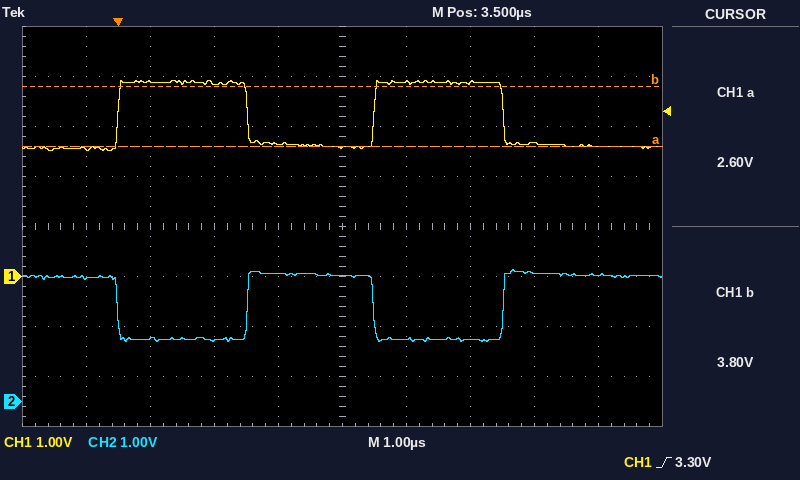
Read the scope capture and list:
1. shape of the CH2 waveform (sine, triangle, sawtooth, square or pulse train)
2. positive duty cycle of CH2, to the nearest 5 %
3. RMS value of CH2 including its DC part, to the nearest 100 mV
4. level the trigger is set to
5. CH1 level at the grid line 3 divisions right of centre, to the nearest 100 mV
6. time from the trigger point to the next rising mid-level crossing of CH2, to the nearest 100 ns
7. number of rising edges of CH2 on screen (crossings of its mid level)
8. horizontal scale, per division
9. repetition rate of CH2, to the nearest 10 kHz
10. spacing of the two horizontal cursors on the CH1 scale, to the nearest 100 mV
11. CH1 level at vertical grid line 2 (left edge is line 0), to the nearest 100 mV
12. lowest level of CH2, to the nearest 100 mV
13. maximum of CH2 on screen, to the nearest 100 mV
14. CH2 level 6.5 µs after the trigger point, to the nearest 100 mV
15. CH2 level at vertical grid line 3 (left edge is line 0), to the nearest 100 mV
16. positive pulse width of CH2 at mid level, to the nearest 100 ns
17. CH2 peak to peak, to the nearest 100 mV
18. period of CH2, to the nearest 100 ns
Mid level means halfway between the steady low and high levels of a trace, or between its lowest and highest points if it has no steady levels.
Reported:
square
50 %
2.0 V
3.30 V
2.7 V
2.0 µs
2
1 µs
250 kHz
1.2 V
3.9 V
1.2 V
2.6 V
2.6 V
1.2 V
2.0 µs
1.4 V
4.0 µs
